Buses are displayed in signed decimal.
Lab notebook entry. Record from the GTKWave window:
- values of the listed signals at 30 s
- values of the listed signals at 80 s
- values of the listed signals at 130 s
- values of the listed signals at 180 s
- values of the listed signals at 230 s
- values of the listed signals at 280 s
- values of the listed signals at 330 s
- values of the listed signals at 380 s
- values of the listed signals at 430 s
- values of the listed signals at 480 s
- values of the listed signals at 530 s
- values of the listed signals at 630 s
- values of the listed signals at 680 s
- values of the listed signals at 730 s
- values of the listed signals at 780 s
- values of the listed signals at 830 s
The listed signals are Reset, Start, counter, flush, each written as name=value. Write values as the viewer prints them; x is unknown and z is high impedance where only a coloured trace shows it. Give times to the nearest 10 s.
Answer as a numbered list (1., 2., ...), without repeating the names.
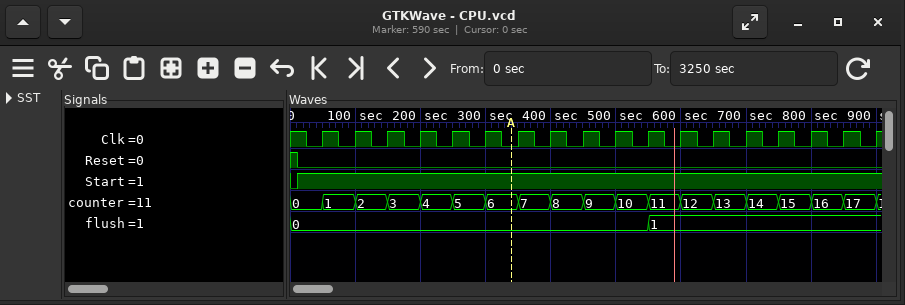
1. Reset=0, Start=1, counter=0, flush=0
2. Reset=0, Start=1, counter=1, flush=0
3. Reset=0, Start=1, counter=2, flush=0
4. Reset=0, Start=1, counter=3, flush=0
5. Reset=0, Start=1, counter=4, flush=0
6. Reset=0, Start=1, counter=5, flush=0
7. Reset=0, Start=1, counter=6, flush=0
8. Reset=0, Start=1, counter=7, flush=0
9. Reset=0, Start=1, counter=8, flush=0
10. Reset=0, Start=1, counter=9, flush=0
11. Reset=0, Start=1, counter=10, flush=0
12. Reset=0, Start=1, counter=12, flush=1
13. Reset=0, Start=1, counter=13, flush=1
14. Reset=0, Start=1, counter=14, flush=1
15. Reset=0, Start=1, counter=15, flush=1
16. Reset=0, Start=1, counter=16, flush=1
